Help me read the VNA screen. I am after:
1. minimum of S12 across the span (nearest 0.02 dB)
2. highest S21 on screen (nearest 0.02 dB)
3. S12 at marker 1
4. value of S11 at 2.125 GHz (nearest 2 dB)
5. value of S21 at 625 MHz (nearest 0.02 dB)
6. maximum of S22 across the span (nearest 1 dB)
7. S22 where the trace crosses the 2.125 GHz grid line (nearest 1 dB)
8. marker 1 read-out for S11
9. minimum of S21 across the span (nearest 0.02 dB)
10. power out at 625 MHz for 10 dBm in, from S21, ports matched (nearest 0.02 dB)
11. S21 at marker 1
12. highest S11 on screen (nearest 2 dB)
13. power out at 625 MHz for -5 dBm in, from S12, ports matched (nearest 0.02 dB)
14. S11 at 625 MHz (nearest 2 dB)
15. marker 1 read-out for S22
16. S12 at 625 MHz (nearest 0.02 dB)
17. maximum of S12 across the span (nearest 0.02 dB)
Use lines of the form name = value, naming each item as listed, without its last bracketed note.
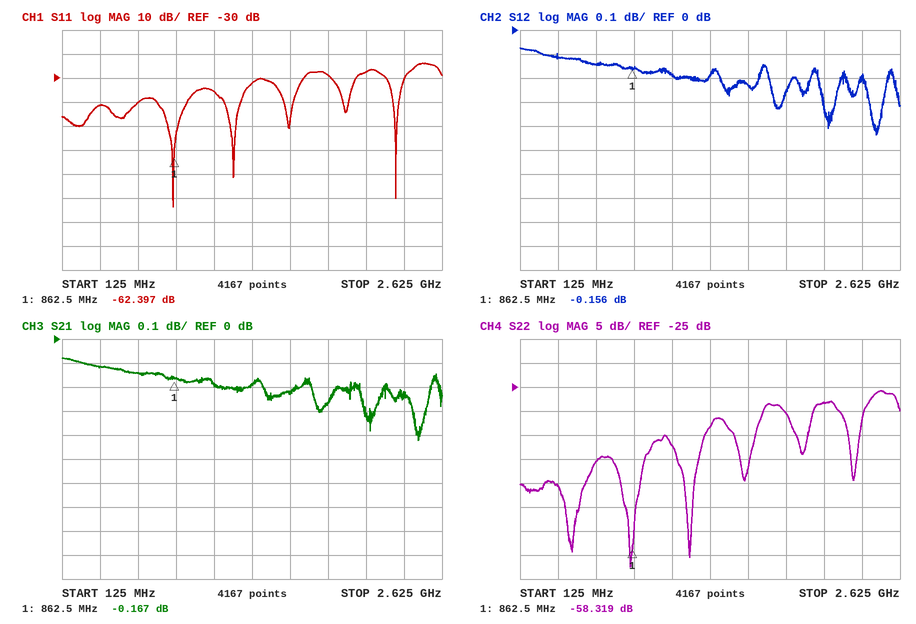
minimum of S12 across the span = -0.44 dB
highest S21 on screen = -0.08 dB
S12 at marker 1 = -0.156 dB
value of S11 at 2.125 GHz = -28 dB
value of S21 at 625 MHz = -0.14 dB
maximum of S22 across the span = -26 dB
S22 where the trace crosses the 2.125 GHz grid line = -28 dB
marker 1 read-out for S11 = -62.397 dB
minimum of S21 across the span = -0.42 dB
power out at 625 MHz for 10 dBm in, from S21, ports matched = 9.86 dBm
S21 at marker 1 = -0.167 dB
highest S11 on screen = -24 dB
power out at 625 MHz for -5 dBm in, from S12, ports matched = -5.14 dBm
S11 at 625 MHz = -40 dB
marker 1 read-out for S22 = -58.319 dB
S12 at 625 MHz = -0.14 dB
maximum of S12 across the span = -0.08 dB
